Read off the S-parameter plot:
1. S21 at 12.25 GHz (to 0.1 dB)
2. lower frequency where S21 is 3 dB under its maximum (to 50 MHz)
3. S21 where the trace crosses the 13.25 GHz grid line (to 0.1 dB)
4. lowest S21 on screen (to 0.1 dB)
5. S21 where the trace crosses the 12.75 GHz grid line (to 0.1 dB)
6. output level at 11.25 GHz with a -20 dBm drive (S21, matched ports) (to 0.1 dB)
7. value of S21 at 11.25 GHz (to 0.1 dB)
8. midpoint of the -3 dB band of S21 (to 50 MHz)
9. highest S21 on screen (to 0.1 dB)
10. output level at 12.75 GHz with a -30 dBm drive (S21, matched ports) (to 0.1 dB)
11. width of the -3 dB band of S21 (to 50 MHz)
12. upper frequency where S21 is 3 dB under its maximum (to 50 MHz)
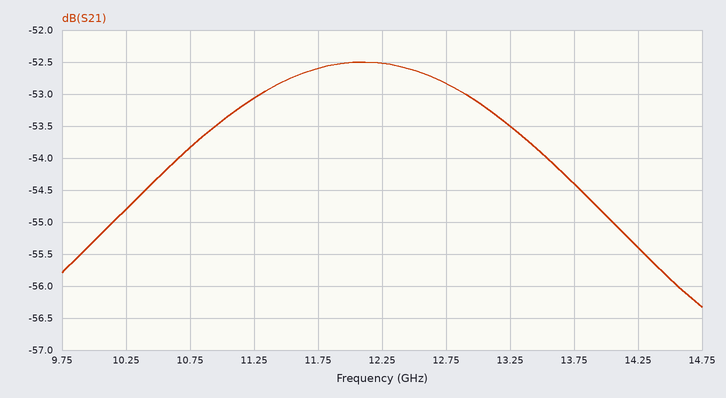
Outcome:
-52.5 dB
9.90 GHz
-53.5 dB
-56.3 dB
-52.8 dB
-73.1 dBm
-53.1 dB
12.10 GHz
-52.5 dB
-82.8 dBm
4.40 GHz
14.30 GHz
